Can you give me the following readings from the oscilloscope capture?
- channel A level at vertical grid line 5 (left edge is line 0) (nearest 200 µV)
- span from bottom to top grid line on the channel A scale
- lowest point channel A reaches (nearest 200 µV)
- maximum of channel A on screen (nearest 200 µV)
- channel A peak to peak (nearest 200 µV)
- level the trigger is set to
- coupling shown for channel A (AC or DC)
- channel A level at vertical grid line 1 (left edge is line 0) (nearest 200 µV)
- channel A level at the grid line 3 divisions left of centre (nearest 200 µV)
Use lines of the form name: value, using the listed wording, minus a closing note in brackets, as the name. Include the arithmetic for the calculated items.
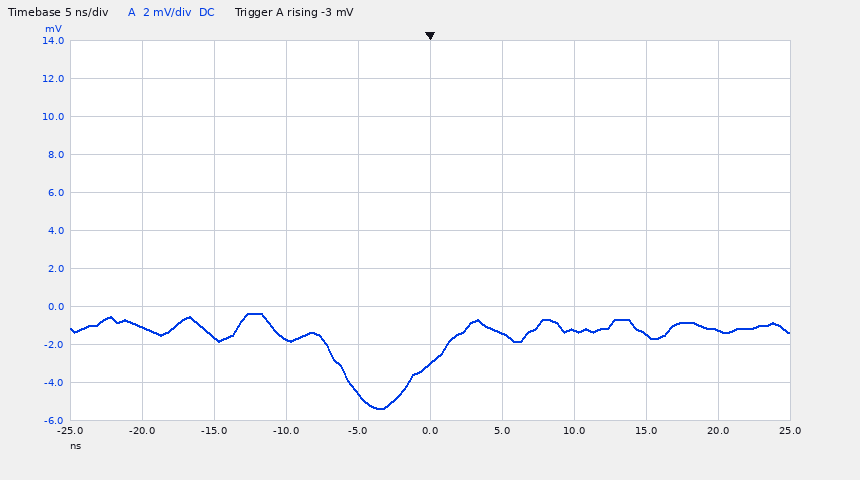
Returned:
channel A level at vertical grid line 5 (left edge is line 0): -3.0 mV
span from bottom to top grid line on the channel A scale: 20 mV
lowest point channel A reaches: -5.4 mV
maximum of channel A on screen: -400 µV
channel A peak to peak: -400 µV − (-5.4 mV) = 5.0 mV
level the trigger is set to: -3 mV
coupling shown for channel A: DC
channel A level at vertical grid line 1 (left edge is line 0): -1.0 mV
channel A level at the grid line 3 divisions left of centre: -1.6 mV
